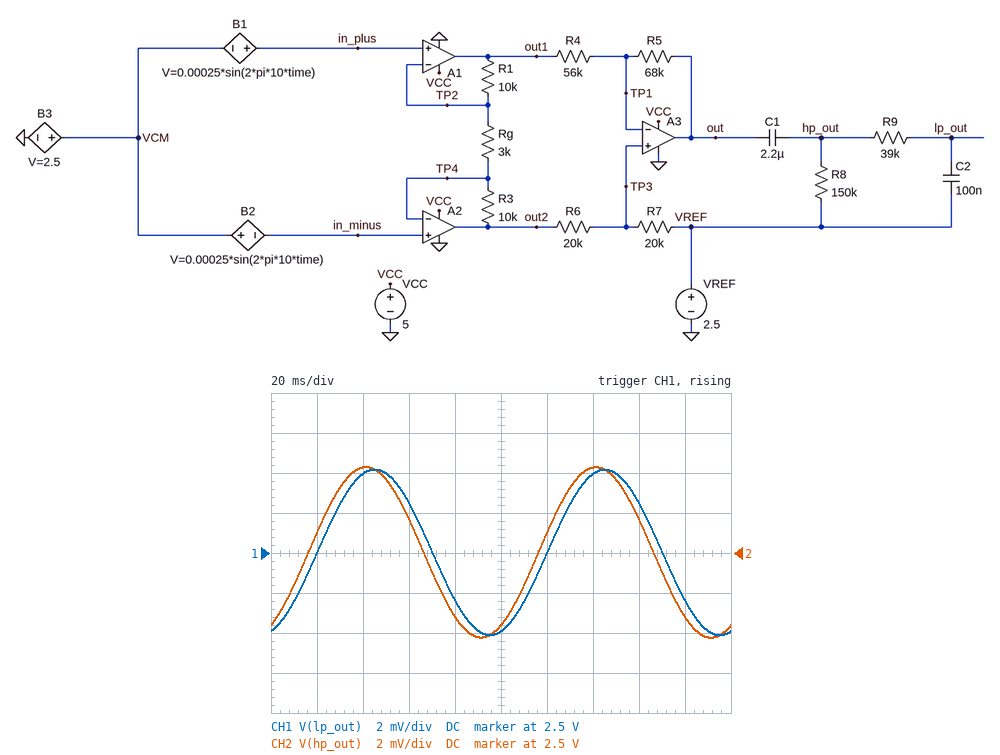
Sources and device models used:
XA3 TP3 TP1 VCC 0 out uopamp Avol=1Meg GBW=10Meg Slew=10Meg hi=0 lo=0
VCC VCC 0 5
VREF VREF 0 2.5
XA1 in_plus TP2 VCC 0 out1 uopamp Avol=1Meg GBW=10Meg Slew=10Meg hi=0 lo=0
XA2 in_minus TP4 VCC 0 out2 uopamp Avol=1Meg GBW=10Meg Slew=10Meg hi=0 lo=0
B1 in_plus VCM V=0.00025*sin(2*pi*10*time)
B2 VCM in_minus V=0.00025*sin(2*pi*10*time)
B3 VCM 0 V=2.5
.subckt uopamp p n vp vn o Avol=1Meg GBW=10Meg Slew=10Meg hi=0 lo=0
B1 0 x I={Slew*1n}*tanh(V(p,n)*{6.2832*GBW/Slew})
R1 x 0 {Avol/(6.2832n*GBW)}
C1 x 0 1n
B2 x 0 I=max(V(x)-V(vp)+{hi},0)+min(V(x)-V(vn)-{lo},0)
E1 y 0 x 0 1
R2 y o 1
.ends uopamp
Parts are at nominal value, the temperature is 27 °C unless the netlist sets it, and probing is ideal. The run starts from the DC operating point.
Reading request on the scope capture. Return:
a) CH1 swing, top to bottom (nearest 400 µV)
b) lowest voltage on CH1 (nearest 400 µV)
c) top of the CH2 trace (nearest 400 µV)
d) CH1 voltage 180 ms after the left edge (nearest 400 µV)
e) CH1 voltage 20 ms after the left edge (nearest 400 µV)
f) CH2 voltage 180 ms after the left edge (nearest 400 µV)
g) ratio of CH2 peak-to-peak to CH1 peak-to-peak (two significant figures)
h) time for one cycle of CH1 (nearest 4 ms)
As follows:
8.4 mV
2.4960 V
2.5044 V
2.4976 V
2.5000 V
2.4968 V
1.0
100 ms
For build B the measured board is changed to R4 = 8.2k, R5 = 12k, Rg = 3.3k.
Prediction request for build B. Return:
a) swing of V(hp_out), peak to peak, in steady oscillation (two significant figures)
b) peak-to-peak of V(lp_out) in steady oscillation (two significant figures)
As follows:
9.1 mV
8.9 mV
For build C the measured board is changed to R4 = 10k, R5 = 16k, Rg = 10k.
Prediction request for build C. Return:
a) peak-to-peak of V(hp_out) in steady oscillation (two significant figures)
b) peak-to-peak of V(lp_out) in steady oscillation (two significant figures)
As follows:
4.2 mV
4.1 mV
